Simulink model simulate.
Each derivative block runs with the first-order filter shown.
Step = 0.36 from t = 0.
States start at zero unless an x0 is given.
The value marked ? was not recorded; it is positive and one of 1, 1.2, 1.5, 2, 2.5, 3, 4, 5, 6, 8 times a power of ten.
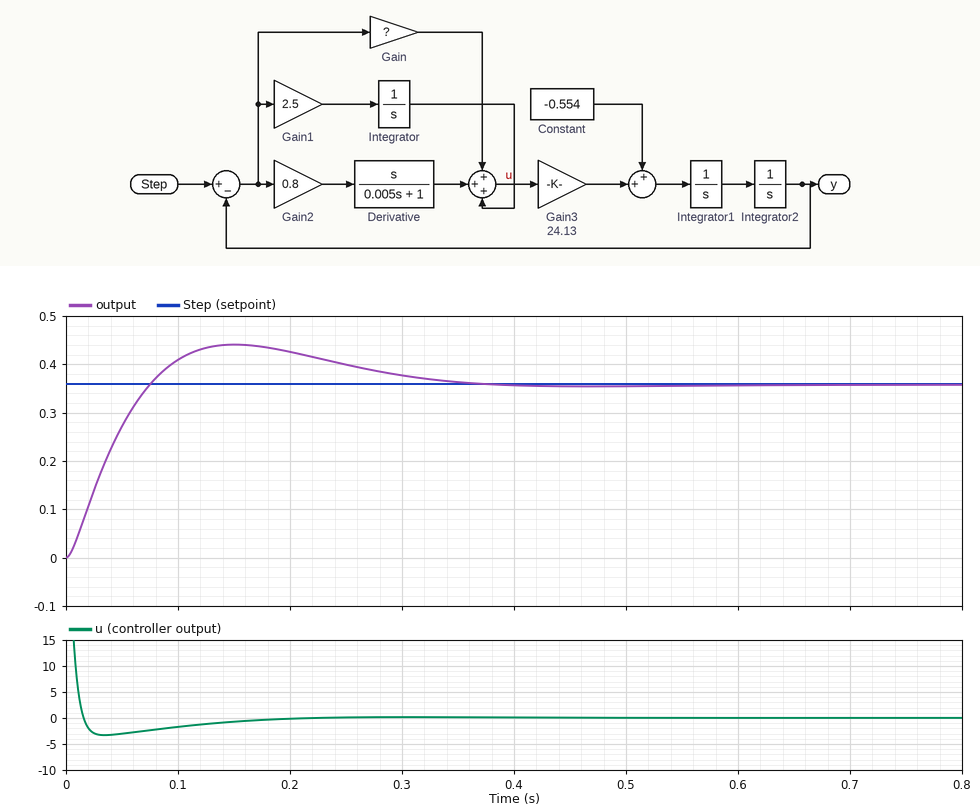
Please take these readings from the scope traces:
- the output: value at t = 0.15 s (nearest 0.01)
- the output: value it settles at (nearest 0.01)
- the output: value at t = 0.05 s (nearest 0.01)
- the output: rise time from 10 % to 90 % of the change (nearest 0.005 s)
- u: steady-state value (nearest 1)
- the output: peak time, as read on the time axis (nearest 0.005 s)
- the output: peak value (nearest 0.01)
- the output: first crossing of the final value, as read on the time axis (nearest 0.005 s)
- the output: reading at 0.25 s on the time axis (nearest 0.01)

0.44
0.36
0.27
0.055 s
0
0.150 s
0.44
0.075 s
0.40
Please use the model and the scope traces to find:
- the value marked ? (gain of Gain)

8
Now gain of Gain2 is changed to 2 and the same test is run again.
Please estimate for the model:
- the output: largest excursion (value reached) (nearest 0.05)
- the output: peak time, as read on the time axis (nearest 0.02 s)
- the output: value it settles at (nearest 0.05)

0.40
0.08 s
0.35
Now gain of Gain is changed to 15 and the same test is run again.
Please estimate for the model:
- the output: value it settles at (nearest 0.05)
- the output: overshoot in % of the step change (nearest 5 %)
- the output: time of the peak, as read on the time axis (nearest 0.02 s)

0.35
30 %
0.12 s
